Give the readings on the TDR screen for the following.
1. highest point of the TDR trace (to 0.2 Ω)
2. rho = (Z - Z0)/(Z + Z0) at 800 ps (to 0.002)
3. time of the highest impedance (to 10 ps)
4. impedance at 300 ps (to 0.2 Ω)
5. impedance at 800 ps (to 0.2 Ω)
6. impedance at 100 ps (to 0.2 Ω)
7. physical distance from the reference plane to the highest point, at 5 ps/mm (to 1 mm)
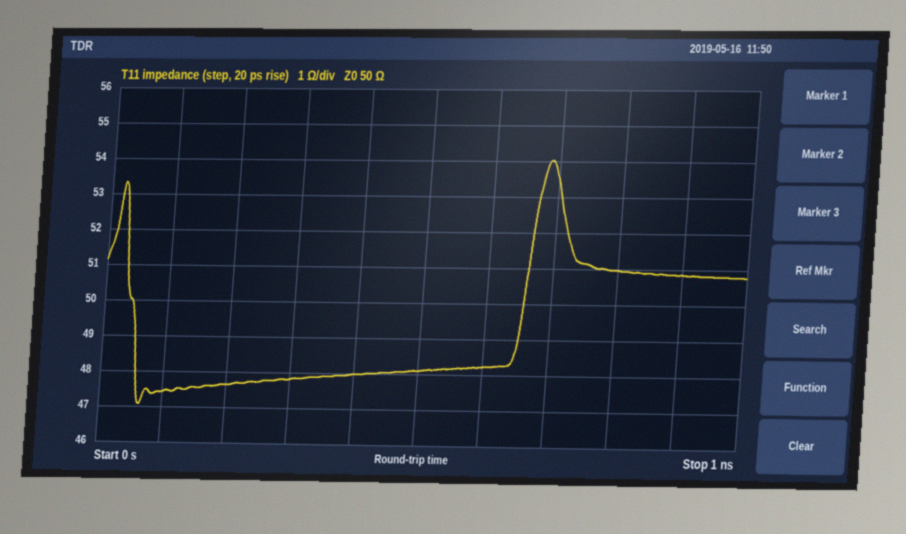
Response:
54.0 Ω
+0.010
690 ps
47.8 Ω
51.0 Ω
47.4 Ω
69 mm
